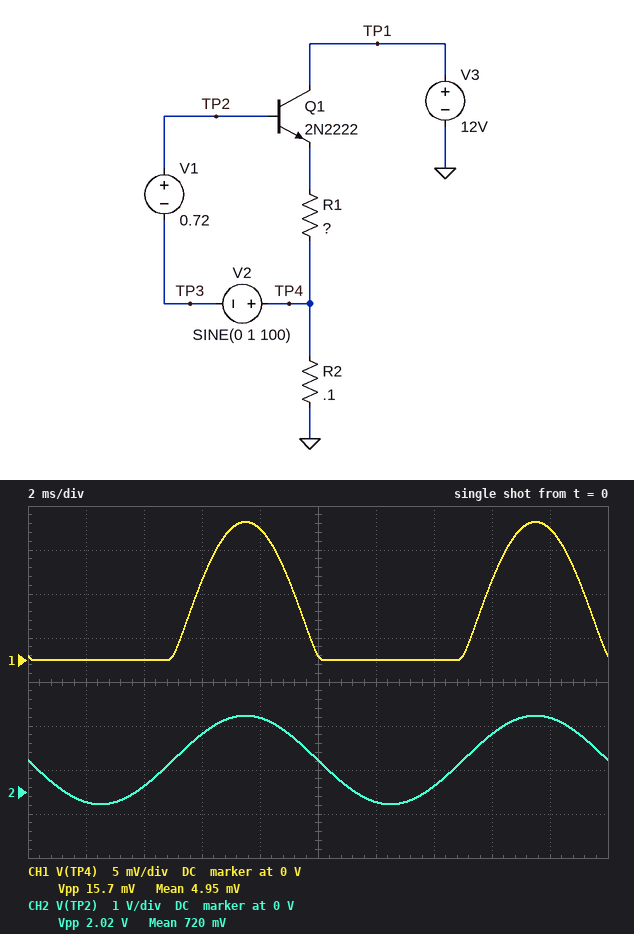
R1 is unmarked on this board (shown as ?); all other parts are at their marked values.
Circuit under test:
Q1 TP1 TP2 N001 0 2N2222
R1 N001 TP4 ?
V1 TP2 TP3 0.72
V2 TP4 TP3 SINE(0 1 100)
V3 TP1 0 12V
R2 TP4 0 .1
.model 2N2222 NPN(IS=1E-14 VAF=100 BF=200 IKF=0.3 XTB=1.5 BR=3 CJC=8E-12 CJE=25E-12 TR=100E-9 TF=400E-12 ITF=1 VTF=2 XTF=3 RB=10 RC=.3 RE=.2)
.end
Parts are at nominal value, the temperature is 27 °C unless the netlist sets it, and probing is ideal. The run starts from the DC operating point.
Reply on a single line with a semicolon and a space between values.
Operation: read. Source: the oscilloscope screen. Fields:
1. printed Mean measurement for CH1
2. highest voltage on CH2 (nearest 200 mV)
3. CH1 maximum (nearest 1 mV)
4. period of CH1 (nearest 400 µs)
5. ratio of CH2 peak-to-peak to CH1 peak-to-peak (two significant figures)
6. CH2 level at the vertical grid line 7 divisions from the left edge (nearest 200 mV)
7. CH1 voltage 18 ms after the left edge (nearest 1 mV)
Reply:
4.95 mV; 1.8 V; 16 mV; 10.0 ms; 130; 200 mV; 15 mV
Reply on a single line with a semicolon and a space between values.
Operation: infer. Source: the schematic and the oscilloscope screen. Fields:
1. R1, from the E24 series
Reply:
5.6 Ω
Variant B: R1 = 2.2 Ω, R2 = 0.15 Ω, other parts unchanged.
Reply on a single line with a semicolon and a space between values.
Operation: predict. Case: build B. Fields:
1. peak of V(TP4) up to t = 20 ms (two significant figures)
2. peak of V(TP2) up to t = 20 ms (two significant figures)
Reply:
53 mV; 1.8 V
